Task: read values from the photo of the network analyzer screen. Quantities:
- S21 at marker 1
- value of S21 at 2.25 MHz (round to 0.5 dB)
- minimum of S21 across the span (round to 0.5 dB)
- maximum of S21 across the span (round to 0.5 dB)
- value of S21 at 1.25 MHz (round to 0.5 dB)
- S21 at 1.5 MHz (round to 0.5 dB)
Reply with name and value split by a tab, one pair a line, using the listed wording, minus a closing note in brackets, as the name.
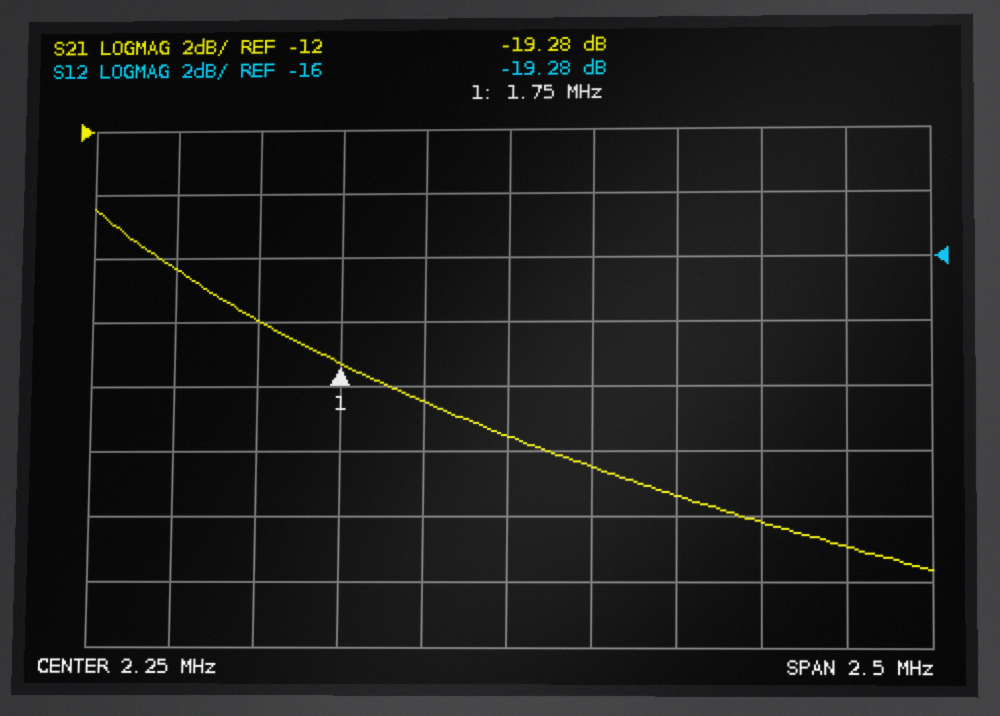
S21 at marker 1	-19.28 dB
value of S21 at 2.25 MHz	-21.5 dB
minimum of S21 across the span	-25.5 dB
maximum of S21 across the span	-14.5 dB
value of S21 at 1.25 MHz	-16.5 dB
S21 at 1.5 MHz	-18.0 dB
